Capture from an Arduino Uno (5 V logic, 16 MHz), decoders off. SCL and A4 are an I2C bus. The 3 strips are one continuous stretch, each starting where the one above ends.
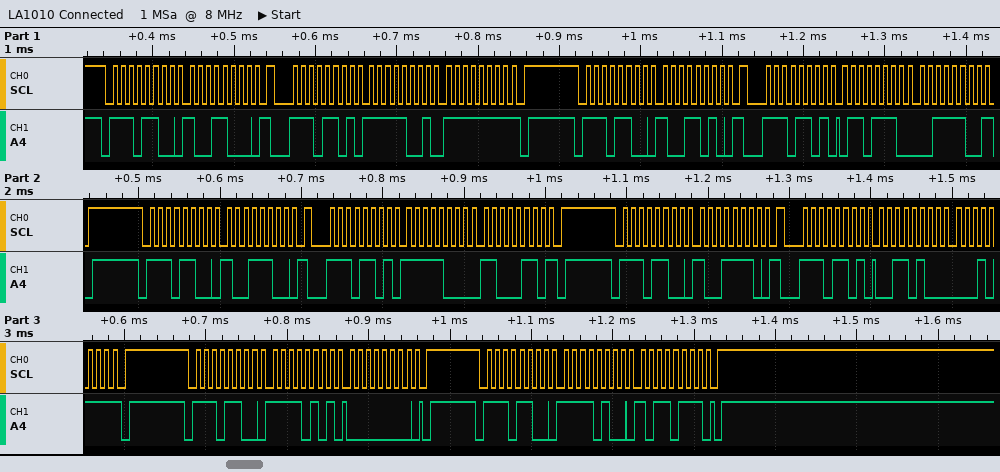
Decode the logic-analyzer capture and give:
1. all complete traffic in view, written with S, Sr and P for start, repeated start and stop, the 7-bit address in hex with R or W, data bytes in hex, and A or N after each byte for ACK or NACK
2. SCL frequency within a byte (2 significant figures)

S 76W A 98 A Sr 76R A F9 A FF N P S 76W A 9A A Sr 76R A 6E A 3C N P S 76W A 9C A Sr 76R A F8 A C6 N P S 76W A 9E A Sr 76R A 34 A 17 N P S 76W A F5 A 00 A P S 76W A F4 A B7 A P
100 kHz
